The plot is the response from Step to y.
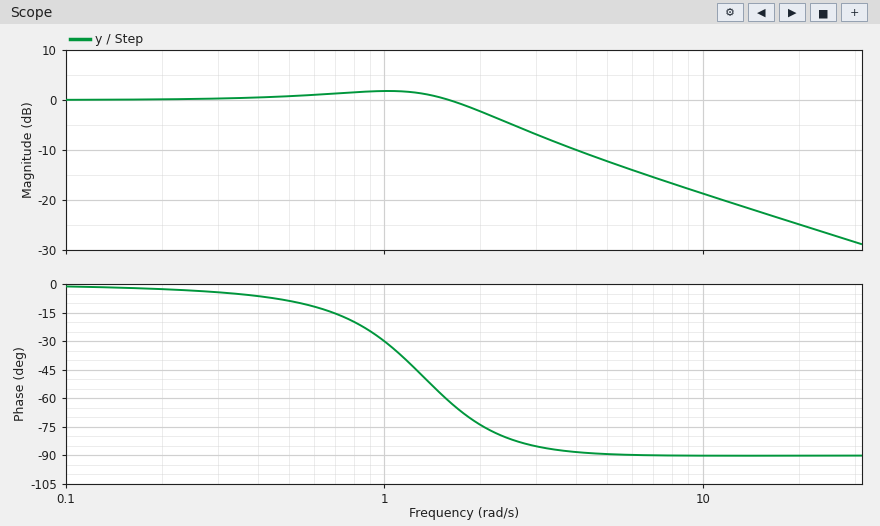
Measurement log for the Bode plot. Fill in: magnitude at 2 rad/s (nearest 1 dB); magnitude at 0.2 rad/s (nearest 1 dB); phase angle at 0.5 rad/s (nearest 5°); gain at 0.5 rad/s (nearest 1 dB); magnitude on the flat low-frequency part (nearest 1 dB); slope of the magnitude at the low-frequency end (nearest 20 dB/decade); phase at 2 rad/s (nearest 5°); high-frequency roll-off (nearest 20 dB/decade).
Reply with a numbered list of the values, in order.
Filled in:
1. -2 dB
2. 0 dB
3. -10°
4. 1 dB
5. 0 dB
6. 0 dB/decade
7. -75°
8. -20 dB/decade
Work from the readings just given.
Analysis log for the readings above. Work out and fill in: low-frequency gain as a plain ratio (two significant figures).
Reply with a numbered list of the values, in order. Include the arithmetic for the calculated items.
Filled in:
1. 10^(0 / 20) = 1.0
